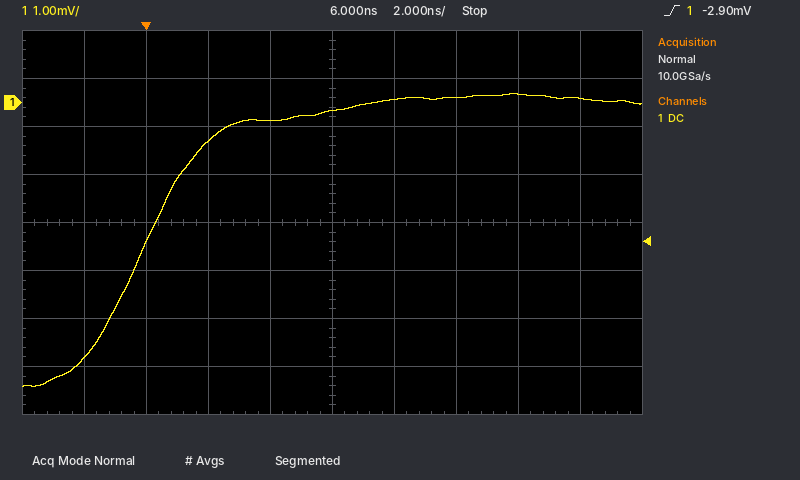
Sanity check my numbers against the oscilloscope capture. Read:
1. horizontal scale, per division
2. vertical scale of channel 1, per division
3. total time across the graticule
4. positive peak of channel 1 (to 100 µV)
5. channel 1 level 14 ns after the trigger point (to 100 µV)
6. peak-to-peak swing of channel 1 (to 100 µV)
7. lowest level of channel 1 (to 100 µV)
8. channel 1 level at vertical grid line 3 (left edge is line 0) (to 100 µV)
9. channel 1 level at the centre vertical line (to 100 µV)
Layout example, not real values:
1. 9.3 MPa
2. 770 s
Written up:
1. 2 ns
2. 1 mV
3. 20 ns
4. 200 µV
5. 100 µV
6. 6.1 mV
7. -5.9 mV
8. -800 µV
9. -200 µV
